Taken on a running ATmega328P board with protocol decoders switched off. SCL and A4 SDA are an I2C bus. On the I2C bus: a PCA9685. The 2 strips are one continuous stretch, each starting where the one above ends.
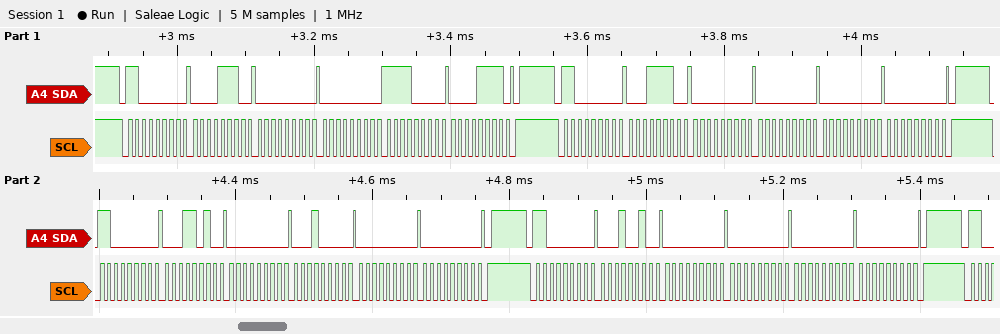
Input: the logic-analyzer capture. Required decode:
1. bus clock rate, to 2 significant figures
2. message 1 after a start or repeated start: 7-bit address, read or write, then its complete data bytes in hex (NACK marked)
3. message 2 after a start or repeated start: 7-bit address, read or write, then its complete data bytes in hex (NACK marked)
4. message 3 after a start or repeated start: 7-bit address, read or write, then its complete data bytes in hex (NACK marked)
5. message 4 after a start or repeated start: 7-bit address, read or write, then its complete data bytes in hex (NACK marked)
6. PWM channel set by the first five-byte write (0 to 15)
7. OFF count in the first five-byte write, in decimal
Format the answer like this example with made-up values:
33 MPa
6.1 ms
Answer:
100 kHz
0x60 write: 0E 00 00 F0 0F
0x60 write: 1E 00 00 00 00
0x60 write: 1A 00 10 00 00
0x60 write: 12 00 00 00 00
2
4080
